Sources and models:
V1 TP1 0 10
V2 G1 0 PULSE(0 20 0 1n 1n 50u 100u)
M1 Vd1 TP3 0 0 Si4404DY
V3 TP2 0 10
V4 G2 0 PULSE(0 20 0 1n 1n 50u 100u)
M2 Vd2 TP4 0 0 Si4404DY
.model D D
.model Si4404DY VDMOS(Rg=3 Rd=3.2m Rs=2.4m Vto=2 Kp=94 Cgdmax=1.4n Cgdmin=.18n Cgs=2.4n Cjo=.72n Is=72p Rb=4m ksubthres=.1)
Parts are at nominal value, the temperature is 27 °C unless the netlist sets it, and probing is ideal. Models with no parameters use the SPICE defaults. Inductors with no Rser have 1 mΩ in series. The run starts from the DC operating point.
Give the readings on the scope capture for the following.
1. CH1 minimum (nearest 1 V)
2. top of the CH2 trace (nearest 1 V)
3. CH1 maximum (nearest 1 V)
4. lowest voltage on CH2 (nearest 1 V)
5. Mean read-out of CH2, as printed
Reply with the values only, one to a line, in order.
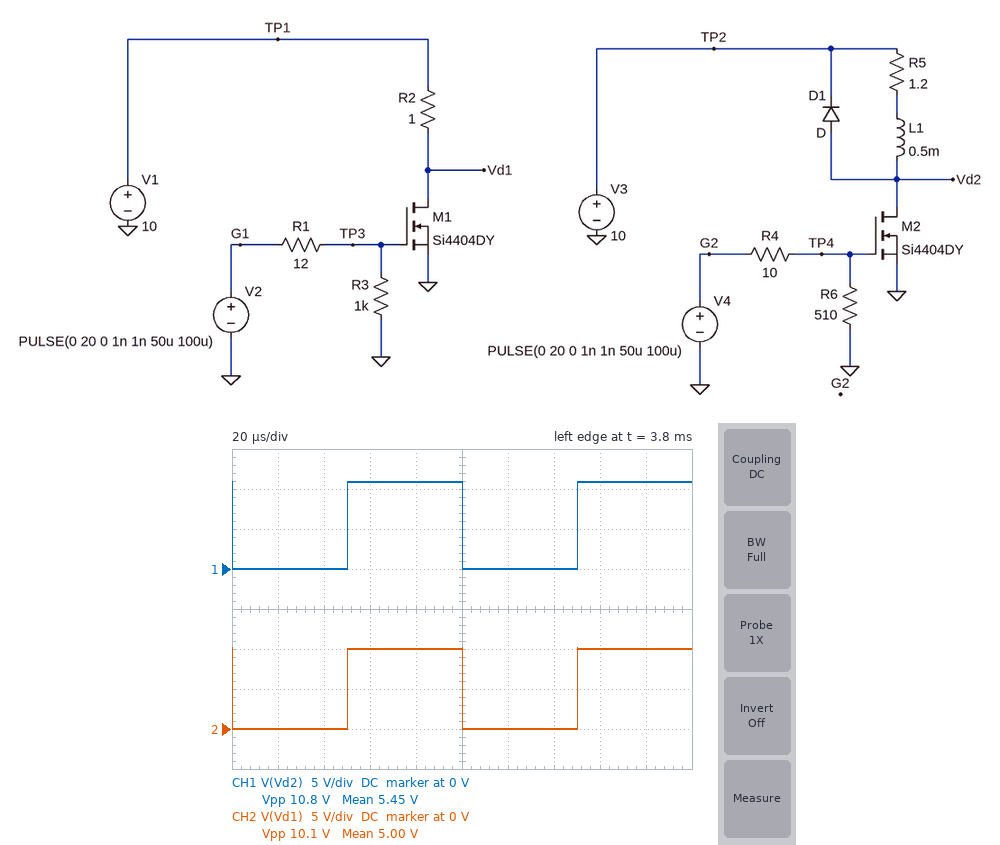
0 V
10 V
11 V
0 V
5.00 V
